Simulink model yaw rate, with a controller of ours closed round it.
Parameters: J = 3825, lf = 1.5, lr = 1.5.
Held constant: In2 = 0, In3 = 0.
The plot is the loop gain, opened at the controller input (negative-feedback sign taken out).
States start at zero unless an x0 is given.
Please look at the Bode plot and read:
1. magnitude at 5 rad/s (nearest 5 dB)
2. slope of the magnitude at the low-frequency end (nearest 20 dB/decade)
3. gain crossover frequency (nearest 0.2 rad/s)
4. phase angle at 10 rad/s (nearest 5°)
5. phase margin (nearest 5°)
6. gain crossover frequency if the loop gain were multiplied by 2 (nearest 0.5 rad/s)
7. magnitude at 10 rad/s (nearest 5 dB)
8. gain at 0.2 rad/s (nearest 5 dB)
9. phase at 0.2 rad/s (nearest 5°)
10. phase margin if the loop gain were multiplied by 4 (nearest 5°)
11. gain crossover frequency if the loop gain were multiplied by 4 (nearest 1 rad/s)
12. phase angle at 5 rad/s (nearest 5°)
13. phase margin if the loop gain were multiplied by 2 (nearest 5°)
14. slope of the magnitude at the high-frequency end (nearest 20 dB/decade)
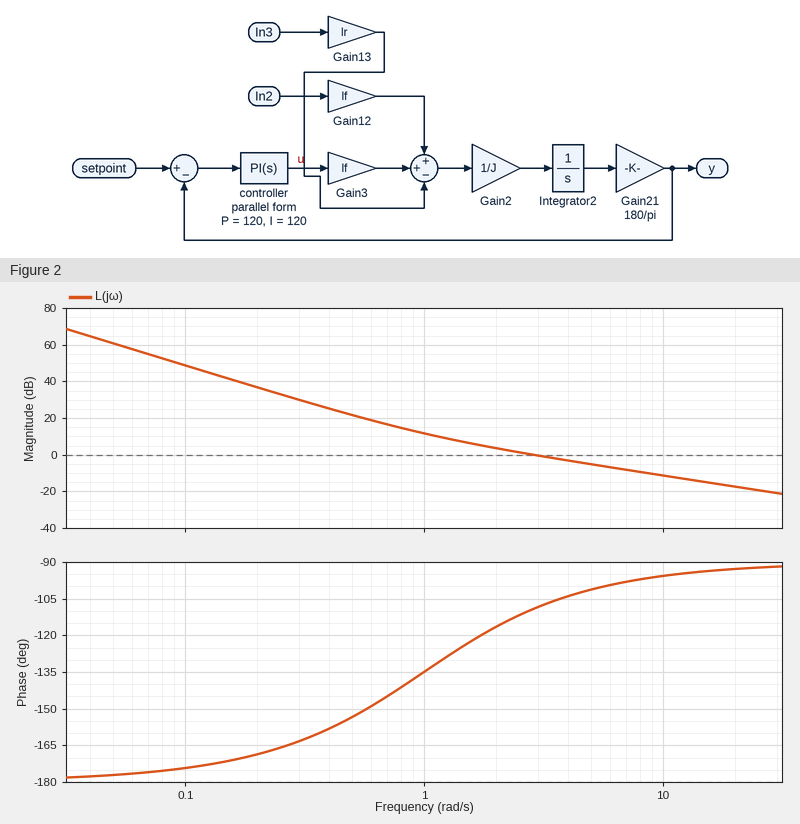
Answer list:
-5 dB
-40 dB/decade
2.8 rad/s
-95°
70°
5.5 rad/s
-10 dB
35 dB
-170°
85°
11 rad/s
-100°
80°
-20 dB/decade
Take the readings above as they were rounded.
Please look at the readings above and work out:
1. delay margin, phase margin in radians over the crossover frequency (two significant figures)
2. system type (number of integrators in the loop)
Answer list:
0.44 s
2
